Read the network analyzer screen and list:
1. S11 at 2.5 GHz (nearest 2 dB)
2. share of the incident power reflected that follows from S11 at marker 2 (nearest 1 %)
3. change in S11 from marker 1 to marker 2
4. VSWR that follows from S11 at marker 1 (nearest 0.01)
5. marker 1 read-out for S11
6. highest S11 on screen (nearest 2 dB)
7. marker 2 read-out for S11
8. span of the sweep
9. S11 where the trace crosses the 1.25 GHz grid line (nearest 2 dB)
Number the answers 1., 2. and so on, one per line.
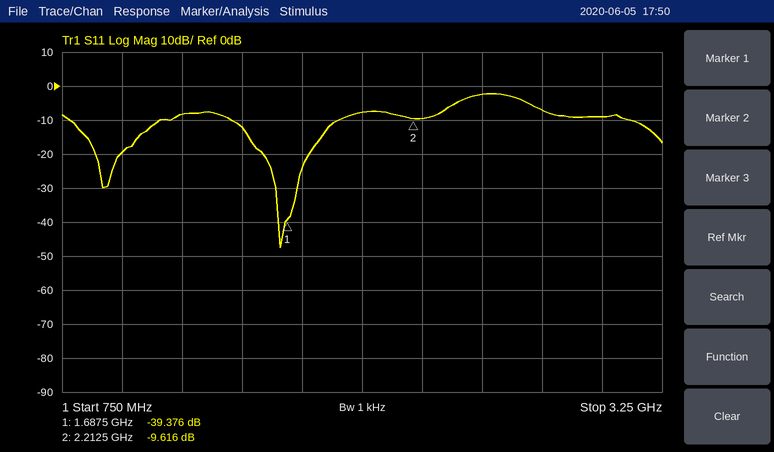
1. -2 dB
2. 11 %
3. 29.760 dB
4. 1.02
5. -39.376 dB
6. -2 dB
7. -9.616 dB
8. 2.5 GHz
9. -8 dB
